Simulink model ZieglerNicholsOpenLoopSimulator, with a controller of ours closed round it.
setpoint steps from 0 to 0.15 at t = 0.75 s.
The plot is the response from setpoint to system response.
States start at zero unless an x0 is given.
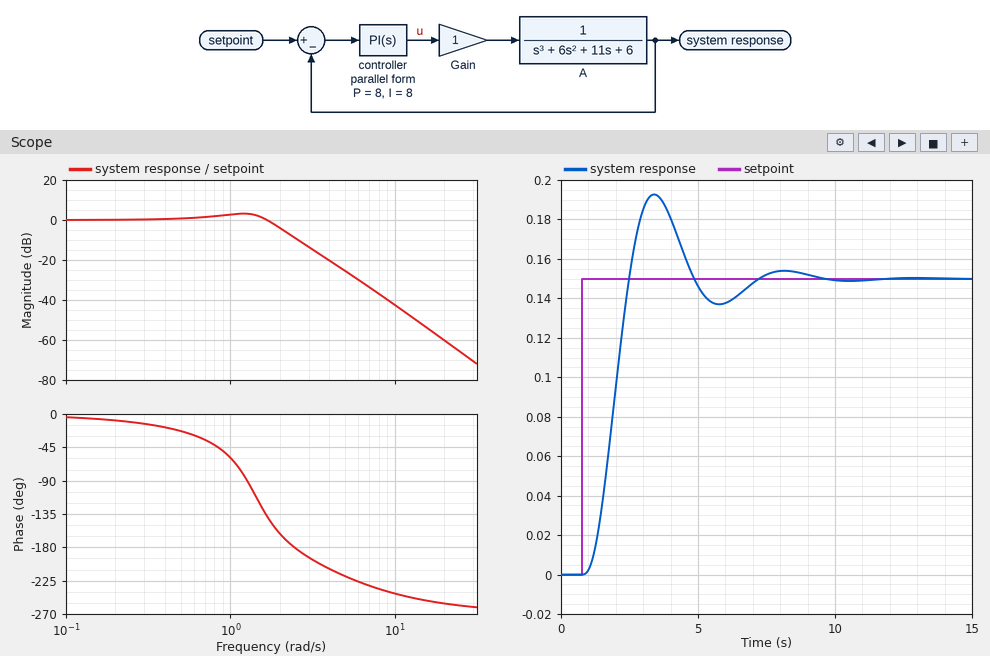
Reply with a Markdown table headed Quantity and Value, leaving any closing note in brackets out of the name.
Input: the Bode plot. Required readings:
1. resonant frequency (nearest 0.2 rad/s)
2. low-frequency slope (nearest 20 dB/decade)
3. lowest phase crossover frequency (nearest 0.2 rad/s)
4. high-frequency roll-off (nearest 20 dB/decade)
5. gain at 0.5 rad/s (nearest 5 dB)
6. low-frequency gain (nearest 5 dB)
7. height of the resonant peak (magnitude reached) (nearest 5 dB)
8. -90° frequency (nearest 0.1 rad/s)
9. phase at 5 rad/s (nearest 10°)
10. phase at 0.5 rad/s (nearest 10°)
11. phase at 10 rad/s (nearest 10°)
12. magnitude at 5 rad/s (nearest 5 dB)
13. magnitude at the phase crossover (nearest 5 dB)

| Quantity | Value |
|---|---|
| resonant frequency | 1.2 rad/s |
| low-frequency slope | 0 dB/decade |
| lowest phase crossover frequency | 2.4 rad/s |
| high-frequency roll-off | -60 dB/decade |
| gain at 0.5 rad/s | 0 dB |
| low-frequency gain | 0 dB |
| height of the resonant peak (magnitude reached) | 5 dB |
| -90° frequency | 1.3 rad/s |
| phase at 5 rad/s | -220° |
| phase at 0.5 rad/s | -20° |
| phase at 10 rad/s | -240° |
| magnitude at 5 rad/s | -25 dB |
| magnitude at the phase crossover | -10 dB |
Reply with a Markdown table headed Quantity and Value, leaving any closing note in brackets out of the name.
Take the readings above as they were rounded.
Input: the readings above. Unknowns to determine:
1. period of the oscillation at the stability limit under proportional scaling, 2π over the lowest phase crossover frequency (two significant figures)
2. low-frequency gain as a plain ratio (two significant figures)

| Quantity | Value |
|---|---|
| period of the oscillation at the stability limit under proportional scaling, 2π over the lowest phase crossover frequency | 2.6 s |
| low-frequency gain as a plain ratio | 1.0 |
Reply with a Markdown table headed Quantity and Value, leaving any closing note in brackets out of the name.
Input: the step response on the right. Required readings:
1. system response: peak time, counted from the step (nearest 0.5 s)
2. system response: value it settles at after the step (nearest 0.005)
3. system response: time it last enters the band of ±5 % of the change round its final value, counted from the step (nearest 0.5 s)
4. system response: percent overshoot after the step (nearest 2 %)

| Quantity | Value |
|---|---|
| system response: peak time, counted from the step | 2.5 s |
| system response: value it settles at after the step | 0.150 |
| system response: time it last enters the band of ±5 % of the change round its final value, counted from the step | 6.0 s |
| system response: percent overshoot after the step | 28 % |
